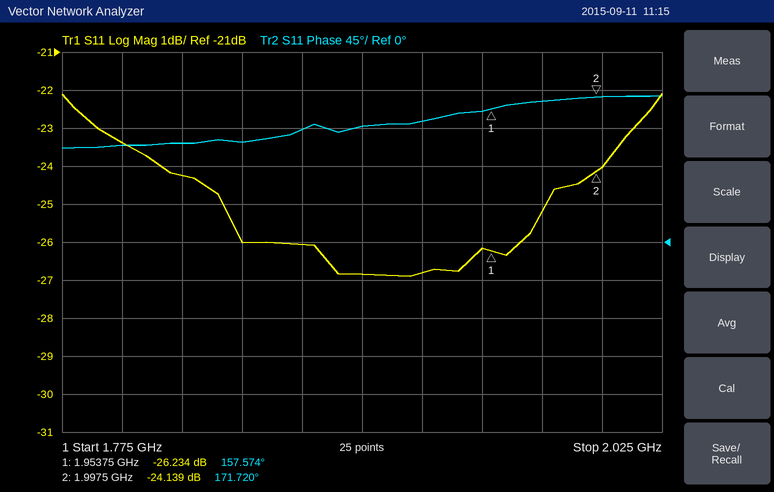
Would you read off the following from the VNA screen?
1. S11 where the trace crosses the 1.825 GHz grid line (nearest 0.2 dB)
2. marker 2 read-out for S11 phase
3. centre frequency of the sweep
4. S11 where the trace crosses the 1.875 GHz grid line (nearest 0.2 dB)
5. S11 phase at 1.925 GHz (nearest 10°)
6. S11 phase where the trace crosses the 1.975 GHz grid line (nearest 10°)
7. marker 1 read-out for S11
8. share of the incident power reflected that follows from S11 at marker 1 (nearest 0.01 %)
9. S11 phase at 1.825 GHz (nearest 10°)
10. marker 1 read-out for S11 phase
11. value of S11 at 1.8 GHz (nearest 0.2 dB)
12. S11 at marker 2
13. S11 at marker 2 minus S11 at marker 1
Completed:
-24.2 dB
171.720°
1.9 GHz
-26.0 dB
140°
170°
-26.234 dB
0.24 %
120°
157.574°
-23.4 dB
-24.139 dB
2.095 dB
